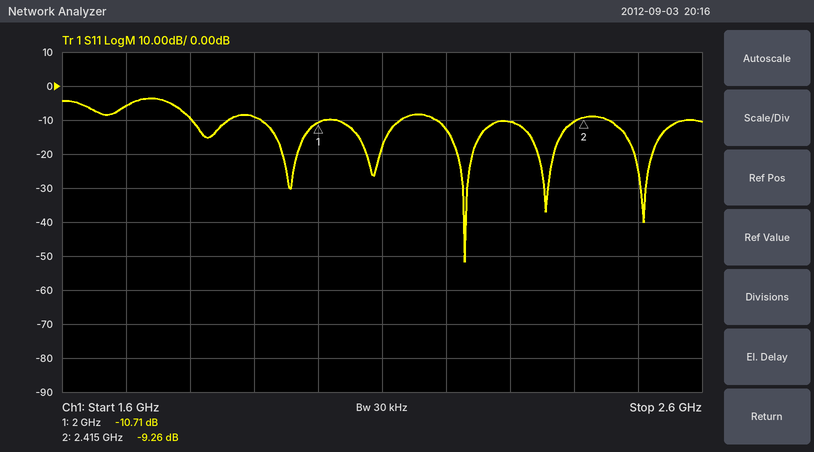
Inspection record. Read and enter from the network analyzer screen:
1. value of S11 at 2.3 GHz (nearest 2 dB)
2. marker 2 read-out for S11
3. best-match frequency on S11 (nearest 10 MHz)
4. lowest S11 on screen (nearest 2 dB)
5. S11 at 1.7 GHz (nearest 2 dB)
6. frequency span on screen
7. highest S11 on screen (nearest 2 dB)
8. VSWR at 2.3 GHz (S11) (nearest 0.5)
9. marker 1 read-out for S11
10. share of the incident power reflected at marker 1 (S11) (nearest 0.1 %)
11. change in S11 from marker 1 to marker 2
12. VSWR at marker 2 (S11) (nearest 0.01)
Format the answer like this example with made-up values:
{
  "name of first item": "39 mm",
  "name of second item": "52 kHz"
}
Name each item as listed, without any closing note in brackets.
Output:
{
  "value of S11 at 2.3 GHz": "-10 dB",
  "marker 2 read-out for S11": "-9.26 dB",
  "best-match frequency on S11": "2.23 GHz",
  "lowest S11 on screen": "-52 dB",
  "S11 at 1.7 GHz": "-6 dB",
  "frequency span on screen": "1 GHz",
  "highest S11 on screen": "-4 dB",
  "VSWR at 2.3 GHz (S11)": "2.0",
  "marker 1 read-out for S11": "-10.71 dB",
  "share of the incident power reflected at marker 1 (S11)": "8.5 %",
  "change in S11 from marker 1 to marker 2": "1.45 dB",
  "VSWR at marker 2 (S11)": "2.05"
}
